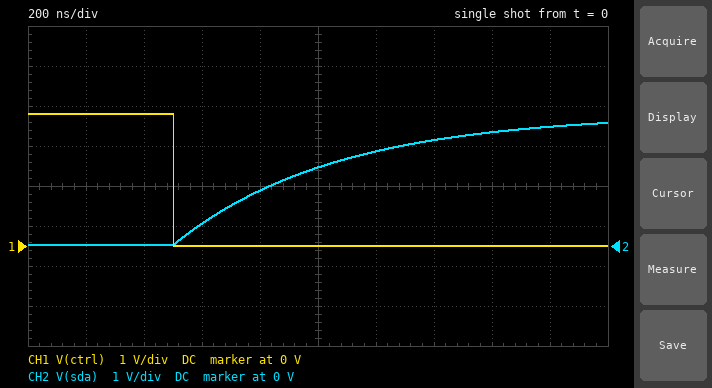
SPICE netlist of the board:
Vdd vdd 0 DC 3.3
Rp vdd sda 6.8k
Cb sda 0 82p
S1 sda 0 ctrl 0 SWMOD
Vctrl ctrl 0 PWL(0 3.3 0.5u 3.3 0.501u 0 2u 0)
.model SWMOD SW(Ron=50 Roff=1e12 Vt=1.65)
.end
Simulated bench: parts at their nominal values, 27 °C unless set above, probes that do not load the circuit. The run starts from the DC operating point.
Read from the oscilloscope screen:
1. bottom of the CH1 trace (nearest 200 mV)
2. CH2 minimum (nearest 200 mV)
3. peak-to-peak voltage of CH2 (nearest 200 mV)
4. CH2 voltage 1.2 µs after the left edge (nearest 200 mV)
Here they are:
0 V
0 V
3.0 V
2.4 V
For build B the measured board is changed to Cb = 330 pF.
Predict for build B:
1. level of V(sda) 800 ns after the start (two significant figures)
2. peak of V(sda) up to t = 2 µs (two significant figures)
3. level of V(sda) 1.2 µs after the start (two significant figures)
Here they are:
430 mV
1.6 V
900 mV
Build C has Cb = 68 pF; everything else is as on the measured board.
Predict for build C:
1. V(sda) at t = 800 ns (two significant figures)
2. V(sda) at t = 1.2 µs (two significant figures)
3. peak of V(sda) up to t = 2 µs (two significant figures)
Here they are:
1.6 V
2.6 V
3.2 V
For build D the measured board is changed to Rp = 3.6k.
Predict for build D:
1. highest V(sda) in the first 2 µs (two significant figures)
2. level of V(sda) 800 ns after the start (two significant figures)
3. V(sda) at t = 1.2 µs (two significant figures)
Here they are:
3.3 V
2.1 V
3.0 V
